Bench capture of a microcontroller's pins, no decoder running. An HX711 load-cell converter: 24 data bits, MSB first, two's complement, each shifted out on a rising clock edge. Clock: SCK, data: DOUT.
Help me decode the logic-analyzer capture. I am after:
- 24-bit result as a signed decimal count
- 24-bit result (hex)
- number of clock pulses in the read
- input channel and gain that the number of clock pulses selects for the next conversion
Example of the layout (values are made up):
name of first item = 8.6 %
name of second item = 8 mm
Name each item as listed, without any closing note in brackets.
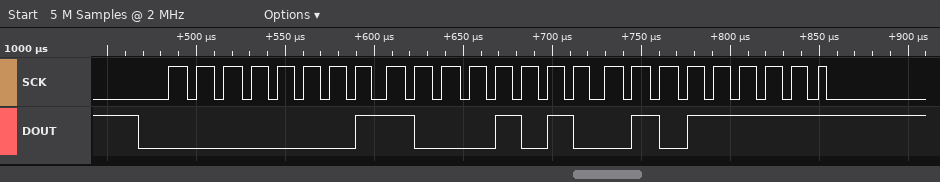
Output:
24-bit result as a signed decimal count = 100959
24-bit result = 0x018A5F
number of clock pulses in the read = 25
input channel and gain that the number of clock pulses selects for the next conversion = channel A, gain 128
